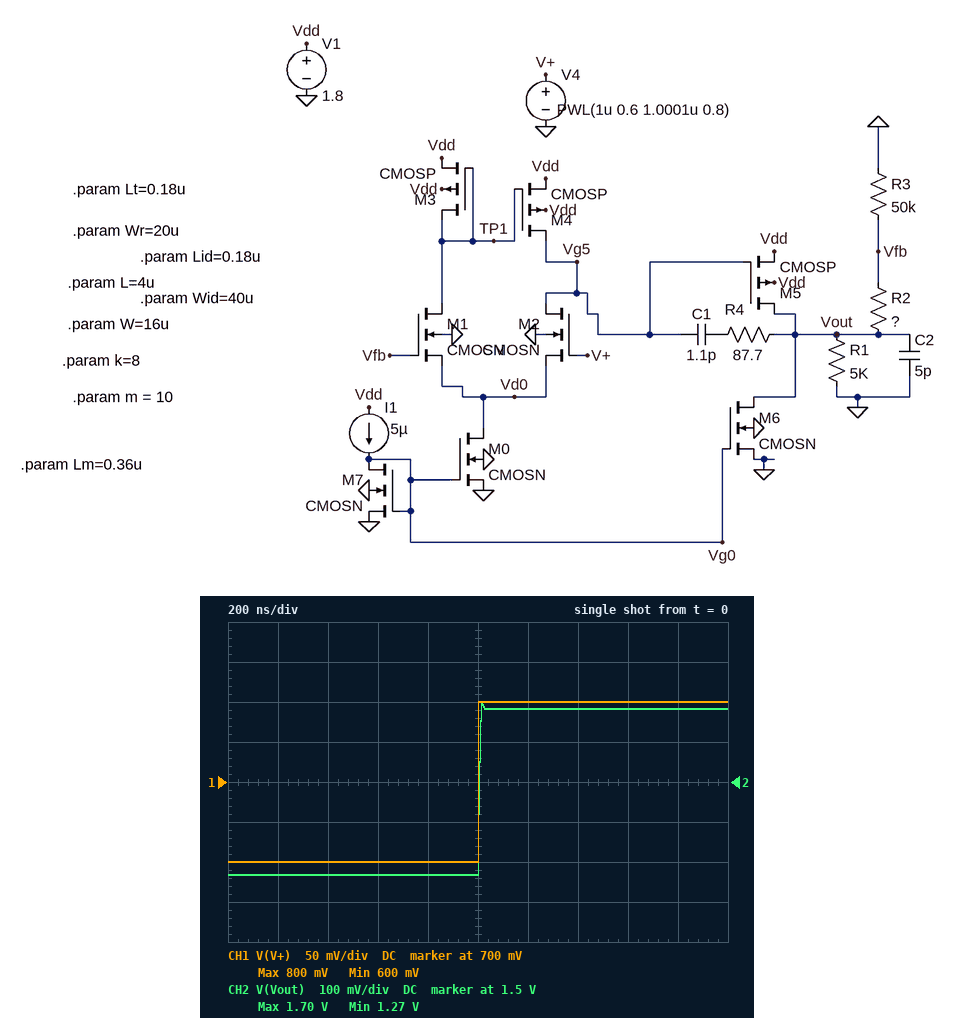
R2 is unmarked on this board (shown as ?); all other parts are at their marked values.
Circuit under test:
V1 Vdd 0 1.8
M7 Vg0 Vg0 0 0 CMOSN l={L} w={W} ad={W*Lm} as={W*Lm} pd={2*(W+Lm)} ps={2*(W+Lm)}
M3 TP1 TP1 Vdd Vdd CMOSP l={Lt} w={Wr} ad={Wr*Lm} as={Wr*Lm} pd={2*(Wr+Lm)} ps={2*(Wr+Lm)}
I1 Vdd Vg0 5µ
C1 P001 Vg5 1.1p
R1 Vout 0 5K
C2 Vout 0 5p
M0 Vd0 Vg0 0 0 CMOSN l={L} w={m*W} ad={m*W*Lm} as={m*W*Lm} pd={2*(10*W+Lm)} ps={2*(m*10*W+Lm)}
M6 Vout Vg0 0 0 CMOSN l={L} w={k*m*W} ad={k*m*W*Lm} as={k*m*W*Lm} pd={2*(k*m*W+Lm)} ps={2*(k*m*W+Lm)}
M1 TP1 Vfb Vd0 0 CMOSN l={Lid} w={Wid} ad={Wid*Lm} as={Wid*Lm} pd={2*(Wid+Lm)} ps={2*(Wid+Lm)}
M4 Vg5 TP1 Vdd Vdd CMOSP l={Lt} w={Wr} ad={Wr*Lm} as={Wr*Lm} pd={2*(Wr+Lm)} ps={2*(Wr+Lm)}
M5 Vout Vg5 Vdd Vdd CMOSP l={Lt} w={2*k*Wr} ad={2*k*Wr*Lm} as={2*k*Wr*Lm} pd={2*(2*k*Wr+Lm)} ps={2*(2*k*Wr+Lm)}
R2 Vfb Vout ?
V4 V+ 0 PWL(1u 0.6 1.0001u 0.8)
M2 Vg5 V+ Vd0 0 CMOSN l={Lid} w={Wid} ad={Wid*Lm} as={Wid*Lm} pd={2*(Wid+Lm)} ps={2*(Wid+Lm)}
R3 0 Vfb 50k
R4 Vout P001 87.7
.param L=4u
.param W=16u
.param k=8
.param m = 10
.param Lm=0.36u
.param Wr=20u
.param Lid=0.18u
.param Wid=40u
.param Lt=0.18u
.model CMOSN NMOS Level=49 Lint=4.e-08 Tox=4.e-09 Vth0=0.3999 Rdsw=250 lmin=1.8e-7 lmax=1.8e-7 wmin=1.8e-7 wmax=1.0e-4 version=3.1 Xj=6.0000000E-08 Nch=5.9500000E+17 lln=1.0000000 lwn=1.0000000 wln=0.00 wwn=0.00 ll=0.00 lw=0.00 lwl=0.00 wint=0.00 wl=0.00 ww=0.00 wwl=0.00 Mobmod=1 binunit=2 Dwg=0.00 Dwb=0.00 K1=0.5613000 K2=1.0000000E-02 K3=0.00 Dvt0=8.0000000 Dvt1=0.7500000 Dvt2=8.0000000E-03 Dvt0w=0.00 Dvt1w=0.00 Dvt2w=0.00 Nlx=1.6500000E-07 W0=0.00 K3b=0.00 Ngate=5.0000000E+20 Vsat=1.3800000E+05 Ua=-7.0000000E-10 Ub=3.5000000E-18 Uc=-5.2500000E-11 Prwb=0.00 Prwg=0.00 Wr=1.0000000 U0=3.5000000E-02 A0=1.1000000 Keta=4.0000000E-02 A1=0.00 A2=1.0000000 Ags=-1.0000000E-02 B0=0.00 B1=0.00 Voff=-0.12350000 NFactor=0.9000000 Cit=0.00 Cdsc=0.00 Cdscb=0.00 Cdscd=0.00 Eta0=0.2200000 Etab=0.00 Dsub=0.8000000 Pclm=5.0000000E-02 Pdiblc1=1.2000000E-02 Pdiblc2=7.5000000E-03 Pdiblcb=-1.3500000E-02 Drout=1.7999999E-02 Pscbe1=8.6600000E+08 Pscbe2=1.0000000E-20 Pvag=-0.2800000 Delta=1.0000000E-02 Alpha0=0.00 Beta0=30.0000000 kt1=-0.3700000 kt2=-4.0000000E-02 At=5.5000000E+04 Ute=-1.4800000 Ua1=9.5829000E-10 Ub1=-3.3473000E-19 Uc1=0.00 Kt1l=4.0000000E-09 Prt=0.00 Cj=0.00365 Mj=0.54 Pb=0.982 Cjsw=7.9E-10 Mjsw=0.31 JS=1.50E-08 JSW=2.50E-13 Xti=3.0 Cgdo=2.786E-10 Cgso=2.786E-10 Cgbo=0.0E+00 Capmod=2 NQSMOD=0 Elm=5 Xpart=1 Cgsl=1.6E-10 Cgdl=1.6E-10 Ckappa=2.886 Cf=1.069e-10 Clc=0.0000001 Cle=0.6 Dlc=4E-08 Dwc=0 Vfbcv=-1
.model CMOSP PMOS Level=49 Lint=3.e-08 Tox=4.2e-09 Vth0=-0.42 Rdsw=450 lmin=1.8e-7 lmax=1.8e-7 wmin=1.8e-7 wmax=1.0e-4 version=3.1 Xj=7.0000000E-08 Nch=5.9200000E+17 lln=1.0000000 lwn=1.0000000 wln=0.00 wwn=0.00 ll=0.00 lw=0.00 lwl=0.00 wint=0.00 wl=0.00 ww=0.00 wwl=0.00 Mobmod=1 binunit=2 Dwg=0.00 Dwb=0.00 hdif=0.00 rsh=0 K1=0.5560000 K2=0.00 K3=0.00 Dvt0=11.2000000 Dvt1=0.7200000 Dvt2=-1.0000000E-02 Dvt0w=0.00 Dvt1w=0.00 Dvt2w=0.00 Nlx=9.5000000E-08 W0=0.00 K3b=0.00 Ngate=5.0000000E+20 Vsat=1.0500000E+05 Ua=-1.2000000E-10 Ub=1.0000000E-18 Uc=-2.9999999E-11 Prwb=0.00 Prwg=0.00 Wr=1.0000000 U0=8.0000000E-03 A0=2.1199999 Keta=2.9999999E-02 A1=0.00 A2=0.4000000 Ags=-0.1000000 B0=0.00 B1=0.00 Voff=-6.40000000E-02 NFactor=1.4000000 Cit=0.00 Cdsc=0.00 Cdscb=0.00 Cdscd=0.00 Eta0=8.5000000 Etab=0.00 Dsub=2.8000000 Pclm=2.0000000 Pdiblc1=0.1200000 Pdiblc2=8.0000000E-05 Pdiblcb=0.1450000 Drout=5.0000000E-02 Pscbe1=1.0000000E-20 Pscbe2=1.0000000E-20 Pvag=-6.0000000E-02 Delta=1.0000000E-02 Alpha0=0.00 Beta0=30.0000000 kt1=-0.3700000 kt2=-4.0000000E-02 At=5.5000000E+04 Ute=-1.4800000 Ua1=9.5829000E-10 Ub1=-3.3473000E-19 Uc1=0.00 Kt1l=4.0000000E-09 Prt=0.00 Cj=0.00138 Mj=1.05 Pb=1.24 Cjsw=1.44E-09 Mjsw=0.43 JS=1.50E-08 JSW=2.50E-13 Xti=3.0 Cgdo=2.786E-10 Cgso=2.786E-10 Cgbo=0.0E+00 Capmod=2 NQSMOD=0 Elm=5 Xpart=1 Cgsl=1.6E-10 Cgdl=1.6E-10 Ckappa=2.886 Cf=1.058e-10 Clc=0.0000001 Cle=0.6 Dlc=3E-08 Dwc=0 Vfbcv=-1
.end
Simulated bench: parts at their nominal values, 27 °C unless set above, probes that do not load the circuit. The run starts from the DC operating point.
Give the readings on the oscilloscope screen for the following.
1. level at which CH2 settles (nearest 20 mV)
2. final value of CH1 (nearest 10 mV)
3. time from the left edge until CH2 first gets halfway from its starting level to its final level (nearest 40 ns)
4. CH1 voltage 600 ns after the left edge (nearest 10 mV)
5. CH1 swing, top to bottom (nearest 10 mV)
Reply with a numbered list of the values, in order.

1. 1.68 V
2. 800 mV
3. 1.00 µs
4. 600 mV
5. 200 mV
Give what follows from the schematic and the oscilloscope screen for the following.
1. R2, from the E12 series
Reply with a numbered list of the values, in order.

1. 56 kΩ
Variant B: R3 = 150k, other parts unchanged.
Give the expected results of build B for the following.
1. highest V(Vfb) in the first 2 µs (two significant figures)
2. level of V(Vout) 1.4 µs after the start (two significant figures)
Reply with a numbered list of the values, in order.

1. 830 mV
2. 1.1 V
